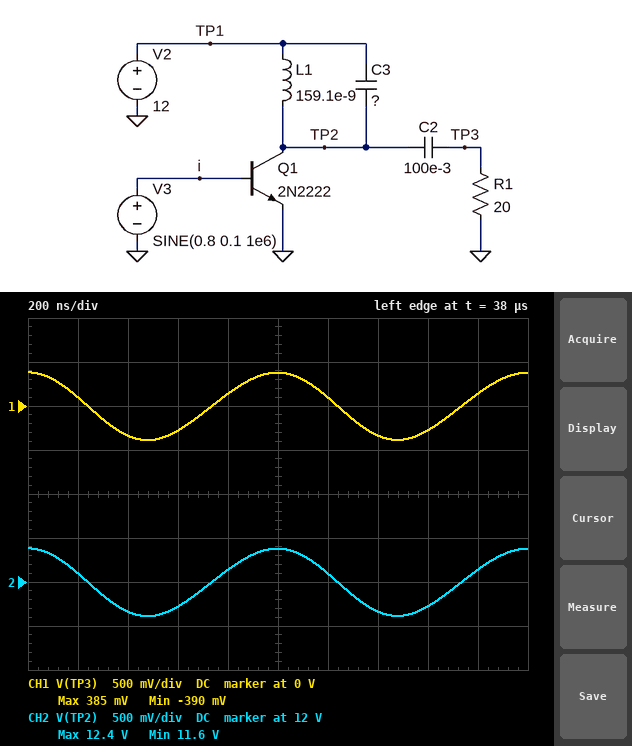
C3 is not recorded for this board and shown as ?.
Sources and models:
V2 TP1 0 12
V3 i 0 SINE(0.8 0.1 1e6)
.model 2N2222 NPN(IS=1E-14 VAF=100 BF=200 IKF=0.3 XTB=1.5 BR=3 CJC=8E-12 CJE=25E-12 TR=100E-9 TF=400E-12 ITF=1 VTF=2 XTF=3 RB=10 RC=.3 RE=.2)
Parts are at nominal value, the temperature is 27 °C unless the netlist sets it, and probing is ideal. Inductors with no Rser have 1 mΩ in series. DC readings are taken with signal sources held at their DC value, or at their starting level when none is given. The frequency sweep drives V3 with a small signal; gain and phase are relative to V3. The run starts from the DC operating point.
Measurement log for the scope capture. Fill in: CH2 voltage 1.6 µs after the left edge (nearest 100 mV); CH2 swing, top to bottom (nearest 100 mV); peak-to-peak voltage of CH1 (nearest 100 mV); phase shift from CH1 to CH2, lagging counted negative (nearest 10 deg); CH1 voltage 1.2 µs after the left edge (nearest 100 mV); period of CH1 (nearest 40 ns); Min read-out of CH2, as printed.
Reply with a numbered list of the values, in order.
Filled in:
1. 11.7 V
2. 800 mV
3. 800 mV
4. 0 deg
5. 100 mV
6. 1.00 µs
7. 11.6 V
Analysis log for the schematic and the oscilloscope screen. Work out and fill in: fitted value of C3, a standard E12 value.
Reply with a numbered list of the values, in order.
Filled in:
1. 220 nF
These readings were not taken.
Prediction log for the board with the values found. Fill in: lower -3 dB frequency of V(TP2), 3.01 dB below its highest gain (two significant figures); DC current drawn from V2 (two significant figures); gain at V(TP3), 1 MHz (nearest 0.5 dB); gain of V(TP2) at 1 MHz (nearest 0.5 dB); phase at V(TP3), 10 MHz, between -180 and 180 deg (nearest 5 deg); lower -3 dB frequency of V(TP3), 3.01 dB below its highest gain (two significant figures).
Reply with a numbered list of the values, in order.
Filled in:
1. 830 kHz
2. 93 mA
3. 12.5 dB
4. 12.5 dB
5. 65 deg
6. 830 kHz
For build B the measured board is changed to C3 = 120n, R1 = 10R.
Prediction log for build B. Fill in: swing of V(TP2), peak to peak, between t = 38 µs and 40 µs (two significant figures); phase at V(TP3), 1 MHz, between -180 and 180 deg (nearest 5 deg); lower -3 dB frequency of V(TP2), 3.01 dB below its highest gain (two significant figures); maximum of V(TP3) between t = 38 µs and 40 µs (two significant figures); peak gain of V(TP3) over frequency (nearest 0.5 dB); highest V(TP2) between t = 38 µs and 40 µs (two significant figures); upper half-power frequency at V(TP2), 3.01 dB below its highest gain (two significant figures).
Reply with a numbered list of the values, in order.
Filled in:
1. 1.1 V
2. -115 deg
3. 1.1 MHz
4. 580 mV
5. 24.0 dB
6. 13 V
7. 1.2 MHz
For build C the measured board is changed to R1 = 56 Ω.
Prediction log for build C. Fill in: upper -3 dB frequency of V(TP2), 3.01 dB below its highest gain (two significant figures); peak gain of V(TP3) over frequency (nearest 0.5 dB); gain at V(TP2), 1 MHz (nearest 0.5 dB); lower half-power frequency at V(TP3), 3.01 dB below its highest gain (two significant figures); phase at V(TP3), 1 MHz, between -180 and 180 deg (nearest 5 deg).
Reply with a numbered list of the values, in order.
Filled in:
1. 860 kHz
2. 38.5 dB
3. 12.5 dB
4. 840 kHz
5. 90 deg
